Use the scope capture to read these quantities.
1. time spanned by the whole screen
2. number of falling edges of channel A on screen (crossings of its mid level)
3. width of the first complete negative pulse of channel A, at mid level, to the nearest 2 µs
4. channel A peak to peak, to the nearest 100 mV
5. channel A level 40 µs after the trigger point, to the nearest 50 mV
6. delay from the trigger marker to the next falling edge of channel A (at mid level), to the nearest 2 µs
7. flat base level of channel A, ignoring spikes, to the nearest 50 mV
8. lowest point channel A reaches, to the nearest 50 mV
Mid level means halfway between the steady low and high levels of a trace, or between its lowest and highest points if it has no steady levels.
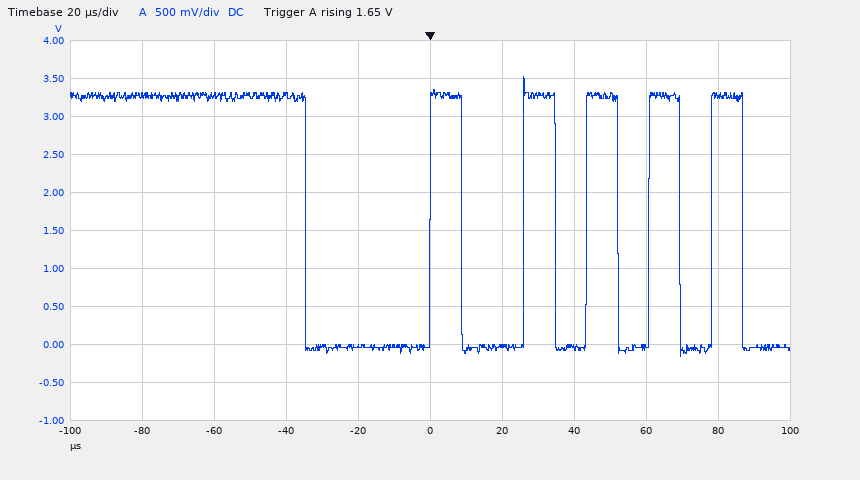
200 µs
6
34 µs
3.70 V
-50 mV
8 µs
-50 mV
-150 mV
